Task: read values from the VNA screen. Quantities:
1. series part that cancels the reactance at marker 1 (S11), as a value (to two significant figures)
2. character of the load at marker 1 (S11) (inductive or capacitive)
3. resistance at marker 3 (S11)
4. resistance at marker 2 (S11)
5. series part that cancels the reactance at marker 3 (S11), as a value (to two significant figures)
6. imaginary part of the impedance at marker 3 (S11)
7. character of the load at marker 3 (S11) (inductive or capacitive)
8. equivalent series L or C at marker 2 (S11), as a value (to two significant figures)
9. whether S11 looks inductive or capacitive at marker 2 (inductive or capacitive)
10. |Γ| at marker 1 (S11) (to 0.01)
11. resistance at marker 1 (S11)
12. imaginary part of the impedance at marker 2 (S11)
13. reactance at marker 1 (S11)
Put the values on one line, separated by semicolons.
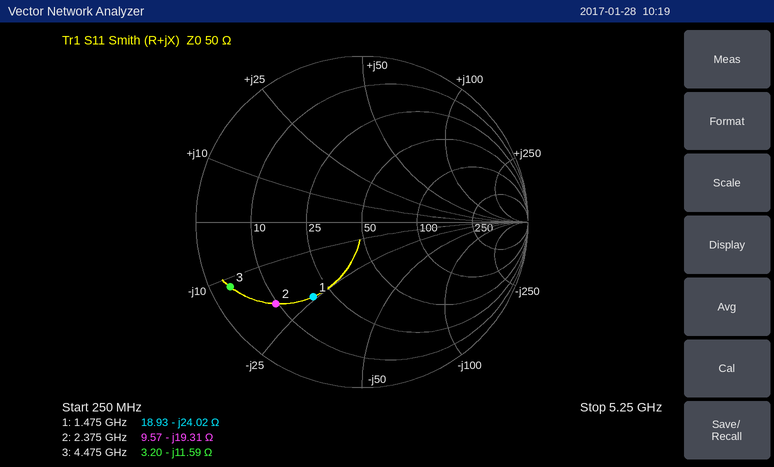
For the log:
2.6 nH; capacitive; 3.20 Ω; 9.57 Ω; 410 pH; -11.59 Ω; capacitive; 3.5 pF; capacitive; 0.54; 18.93 Ω; -19.31 Ω; -24.02 Ω
